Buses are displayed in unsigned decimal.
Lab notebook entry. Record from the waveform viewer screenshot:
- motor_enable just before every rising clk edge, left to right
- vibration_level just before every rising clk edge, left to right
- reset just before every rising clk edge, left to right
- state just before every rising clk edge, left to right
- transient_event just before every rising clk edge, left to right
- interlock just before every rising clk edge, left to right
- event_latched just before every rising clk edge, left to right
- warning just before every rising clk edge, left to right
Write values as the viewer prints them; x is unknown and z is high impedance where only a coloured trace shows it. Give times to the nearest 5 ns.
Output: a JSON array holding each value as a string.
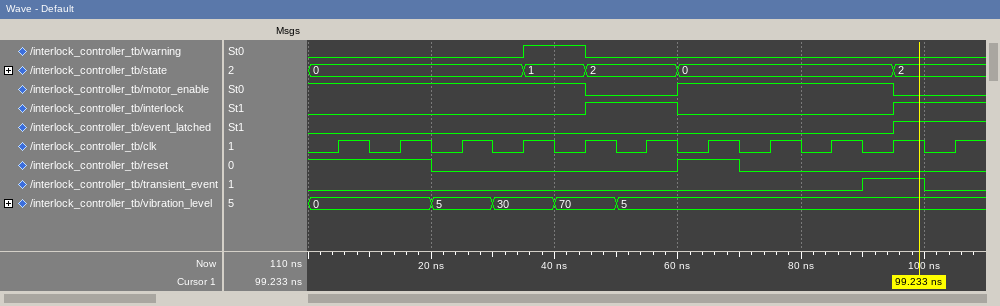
["1 1 1 1 1 0 1 1 1 1 0", "0, 0, 5, 30, 70, 5, 5, 5, 5, 5, 5", "1 1 0 0 0 0 1 0 0 0 0", "0, 0, 0, 0, 1, 2, 0, 0, 0, 0, 2", "0 0 0 0 0 0 0 0 0 1 0", "0 0 0 0 0 1 0 0 0 0 1", "0 0 0 0 0 0 0 0 0 0 1", "0 0 0 0 1 0 0 0 0 0 0"]
